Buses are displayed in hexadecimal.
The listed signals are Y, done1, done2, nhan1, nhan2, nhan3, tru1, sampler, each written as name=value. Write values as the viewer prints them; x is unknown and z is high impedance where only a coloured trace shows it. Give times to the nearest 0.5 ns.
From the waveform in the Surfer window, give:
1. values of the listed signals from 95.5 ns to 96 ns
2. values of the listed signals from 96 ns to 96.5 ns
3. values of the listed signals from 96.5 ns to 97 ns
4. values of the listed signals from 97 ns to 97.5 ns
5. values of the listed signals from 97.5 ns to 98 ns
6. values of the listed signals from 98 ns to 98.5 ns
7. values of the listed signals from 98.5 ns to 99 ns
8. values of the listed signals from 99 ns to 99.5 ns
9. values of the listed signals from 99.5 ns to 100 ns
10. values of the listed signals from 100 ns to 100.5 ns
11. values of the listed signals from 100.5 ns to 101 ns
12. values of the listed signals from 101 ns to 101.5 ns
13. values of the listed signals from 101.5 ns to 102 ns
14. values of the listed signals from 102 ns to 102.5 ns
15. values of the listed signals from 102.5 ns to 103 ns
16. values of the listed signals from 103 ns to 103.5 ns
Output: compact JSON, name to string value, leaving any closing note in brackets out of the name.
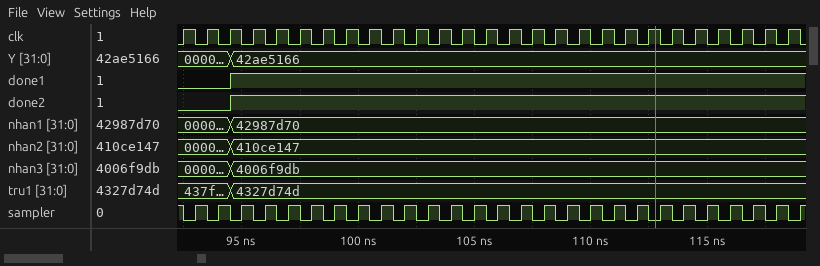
{"values of the listed signals from 95.5 ns to 96 ns": "Y=42ae5166, done1=1, done2=1, nhan1=42987d70, nhan2=410ce147, nhan3=4006f9db, tru1=4327d74d, sampler=0", "values of the listed signals from 96 ns to 96.5 ns": "Y=42ae5166, done1=1, done2=1, nhan1=42987d70, nhan2=410ce147, nhan3=4006f9db, tru1=4327d74d, sampler=1", "values of the listed signals from 96.5 ns to 97 ns": "Y=42ae5166, done1=1, done2=1, nhan1=42987d70, nhan2=410ce147, nhan3=4006f9db, tru1=4327d74d, sampler=0", "values of the listed signals from 97 ns to 97.5 ns": "Y=42ae5166, done1=1, done2=1, nhan1=42987d70, nhan2=410ce147, nhan3=4006f9db, tru1=4327d74d, sampler=1", "values of the listed signals from 97.5 ns to 98 ns": "Y=42ae5166, done1=1, done2=1, nhan1=42987d70, nhan2=410ce147, nhan3=4006f9db, tru1=4327d74d, sampler=0", "values of the listed signals from 98 ns to 98.5 ns": "Y=42ae5166, done1=1, done2=1, nhan1=42987d70, nhan2=410ce147, nhan3=4006f9db, tru1=4327d74d, sampler=1", "values of the listed signals from 98.5 ns to 99 ns": "Y=42ae5166, done1=1, done2=1, nhan1=42987d70, nhan2=410ce147, nhan3=4006f9db, tru1=4327d74d, sampler=0", "values of the listed signals from 99 ns to 99.5 ns": "Y=42ae5166, done1=1, done2=1, nhan1=42987d70, nhan2=410ce147, nhan3=4006f9db, tru1=4327d74d, sampler=1", "values of the listed signals from 99.5 ns to 100 ns": "Y=42ae5166, done1=1, done2=1, nhan1=42987d70, nhan2=410ce147, nhan3=4006f9db, tru1=4327d74d, sampler=0", "values of the listed signals from 100 ns to 100.5 ns": "Y=42ae5166, done1=1, done2=1, nhan1=42987d70, nhan2=410ce147, nhan3=4006f9db, tru1=4327d74d, sampler=1", "values of the listed signals from 100.5 ns to 101 ns": "Y=42ae5166, done1=1, done2=1, nhan1=42987d70, nhan2=410ce147, nhan3=4006f9db, tru1=4327d74d, sampler=0", "values of the listed signals from 101 ns to 101.5 ns": "Y=42ae5166, done1=1, done2=1, nhan1=42987d70, nhan2=410ce147, nhan3=4006f9db, tru1=4327d74d, sampler=1", "values of the listed signals from 101.5 ns to 102 ns": "Y=42ae5166, done1=1, done2=1, nhan1=42987d70, nhan2=410ce147, nhan3=4006f9db, tru1=4327d74d, sampler=0", "values of the listed signals from 102 ns to 102.5 ns": "Y=42ae5166, done1=1, done2=1, nhan1=42987d70, nhan2=410ce147, nhan3=4006f9db, tru1=4327d74d, sampler=1", "values of the listed signals from 102.5 ns to 103 ns": "Y=42ae5166, done1=1, done2=1, nhan1=42987d70, nhan2=410ce147, nhan3=4006f9db, tru1=4327d74d, sampler=0", "values of the listed signals from 103 ns to 103.5 ns": "Y=42ae5166, done1=1, done2=1, nhan1=42987d70, nhan2=410ce147, nhan3=4006f9db, tru1=4327d74d, sampler=1"}
